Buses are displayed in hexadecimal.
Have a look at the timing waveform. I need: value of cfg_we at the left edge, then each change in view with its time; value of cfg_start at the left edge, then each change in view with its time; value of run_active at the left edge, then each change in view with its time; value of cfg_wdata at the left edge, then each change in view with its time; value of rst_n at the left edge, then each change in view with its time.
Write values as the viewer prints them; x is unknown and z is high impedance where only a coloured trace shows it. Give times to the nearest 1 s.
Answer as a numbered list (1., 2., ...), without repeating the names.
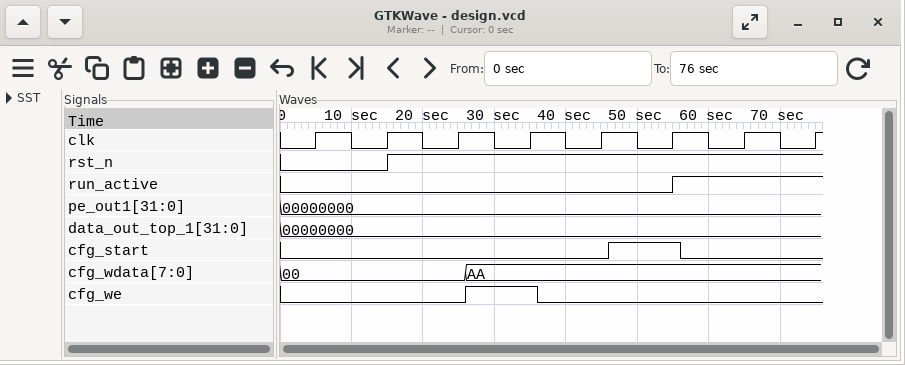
1. 0, 1 at 26 s, 0 at 36 s
2. 0, 1 at 46 s, 0 at 56 s
3. 0, 1 at 55 s
4. 00, AA at 26 s
5. 0, 1 at 15 s
